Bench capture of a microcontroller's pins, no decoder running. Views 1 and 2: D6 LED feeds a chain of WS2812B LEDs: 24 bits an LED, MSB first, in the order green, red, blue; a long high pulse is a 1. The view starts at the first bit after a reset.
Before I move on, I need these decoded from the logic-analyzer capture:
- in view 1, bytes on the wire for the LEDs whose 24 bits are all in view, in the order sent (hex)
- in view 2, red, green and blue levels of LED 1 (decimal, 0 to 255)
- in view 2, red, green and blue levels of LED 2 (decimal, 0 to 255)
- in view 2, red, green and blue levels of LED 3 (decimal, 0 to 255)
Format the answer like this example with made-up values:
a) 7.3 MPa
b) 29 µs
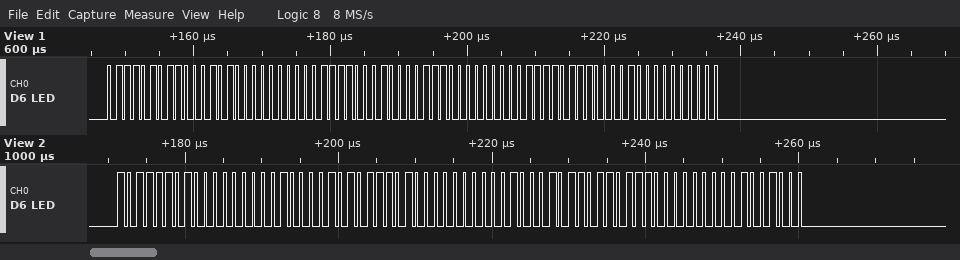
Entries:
a) 75 8A 00 78 87 00 7B 84 00
b) 0, 189, 66
c) 0, 186, 69
d) 0, 183, 72
